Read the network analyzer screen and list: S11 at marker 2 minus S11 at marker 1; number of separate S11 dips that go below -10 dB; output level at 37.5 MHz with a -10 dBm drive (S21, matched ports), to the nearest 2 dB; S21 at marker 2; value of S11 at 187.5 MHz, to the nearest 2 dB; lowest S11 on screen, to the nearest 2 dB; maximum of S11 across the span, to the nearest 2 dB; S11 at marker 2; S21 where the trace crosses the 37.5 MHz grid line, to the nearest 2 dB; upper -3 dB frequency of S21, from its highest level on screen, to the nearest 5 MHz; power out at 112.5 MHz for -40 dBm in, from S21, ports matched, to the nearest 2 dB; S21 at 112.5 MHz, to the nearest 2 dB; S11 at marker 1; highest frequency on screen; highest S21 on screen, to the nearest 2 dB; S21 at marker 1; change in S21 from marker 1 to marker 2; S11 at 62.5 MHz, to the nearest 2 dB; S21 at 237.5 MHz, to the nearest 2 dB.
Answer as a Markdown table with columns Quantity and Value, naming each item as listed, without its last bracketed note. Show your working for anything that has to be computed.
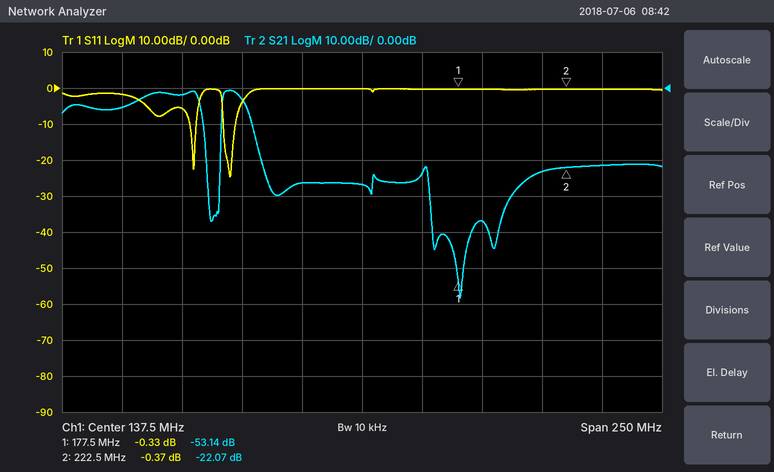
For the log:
| Quantity | Value |
|---|---|
| S11 at marker 2 minus S11 at marker 1 | -0.37 − (-0.33) = -0.04 dB |
| number of separate S11 dips that go below -10 dB | 2 |
| output level at 37.5 MHz with a -10 dBm drive (S21, matched ports), to the nearest 2 dB | -10 dBm + (-6 dB) = -16 dBm |
| S21 at marker 2 | -22.07 dB |
| value of S11 at 187.5 MHz, to the nearest 2 dB | 0 dB |
| lowest S11 on screen, to the nearest 2 dB | -24 dB |
| maximum of S11 across the span, to the nearest 2 dB | 0 dB |
| S11 at marker 2 | -0.37 dB |
| S21 where the trace crosses the 37.5 MHz grid line, to the nearest 2 dB | -6 dB |
| upper -3 dB frequency of S21, from its highest level on screen, to the nearest 5 MHz | 90 MHz |
| power out at 112.5 MHz for -40 dBm in, from S21, ports matched, to the nearest 2 dB | -40 dBm + (-26 dB) = -66 dBm |
| S21 at 112.5 MHz, to the nearest 2 dB | -26 dB |
| S11 at marker 1 | -0.33 dB |
| highest frequency on screen | 262.5 MHz |
| highest S21 on screen, to the nearest 2 dB | 0 dB |
| S21 at marker 1 | -53.14 dB |
| change in S21 from marker 1 to marker 2 | -22.07 − (-53.14) = 31.07 dB |
| S11 at 62.5 MHz, to the nearest 2 dB | -6 dB |
| S21 at 237.5 MHz, to the nearest 2 dB | -22 dB |
